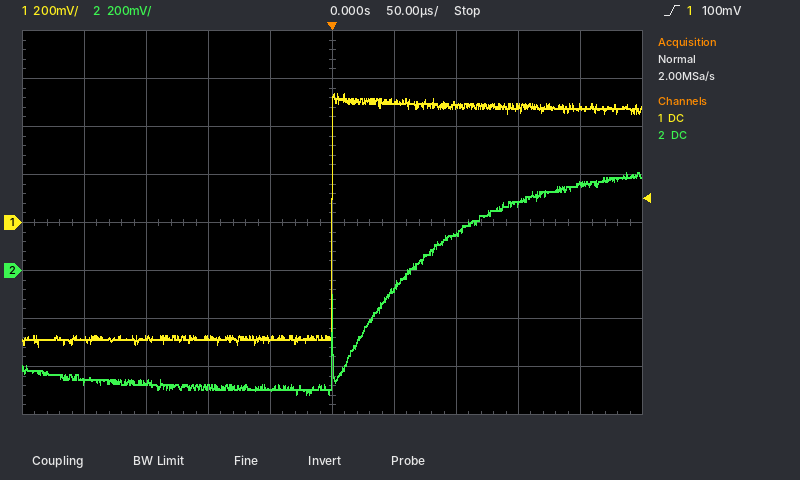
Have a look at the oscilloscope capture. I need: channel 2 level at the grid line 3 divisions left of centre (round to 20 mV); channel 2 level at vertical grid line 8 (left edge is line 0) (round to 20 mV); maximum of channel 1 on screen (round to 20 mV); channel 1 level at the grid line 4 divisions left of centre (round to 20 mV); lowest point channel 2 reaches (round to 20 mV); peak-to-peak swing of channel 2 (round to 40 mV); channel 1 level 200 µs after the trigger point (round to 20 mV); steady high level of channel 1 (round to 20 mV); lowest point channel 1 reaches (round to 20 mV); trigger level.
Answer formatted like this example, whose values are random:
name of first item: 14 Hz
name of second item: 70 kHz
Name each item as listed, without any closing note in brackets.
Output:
channel 2 level at the grid line 3 divisions left of centre: -460 mV
channel 2 level at vertical grid line 8 (left edge is line 0): 280 mV
maximum of channel 1 on screen: 540 mV
channel 1 level at the grid line 4 divisions left of centre: -480 mV
lowest point channel 2 reaches: -520 mV
peak-to-peak swing of channel 2: 920 mV
channel 1 level 200 µs after the trigger point: 480 mV
steady high level of channel 1: 480 mV
lowest point channel 1 reaches: -520 mV
trigger level: 100 mV
